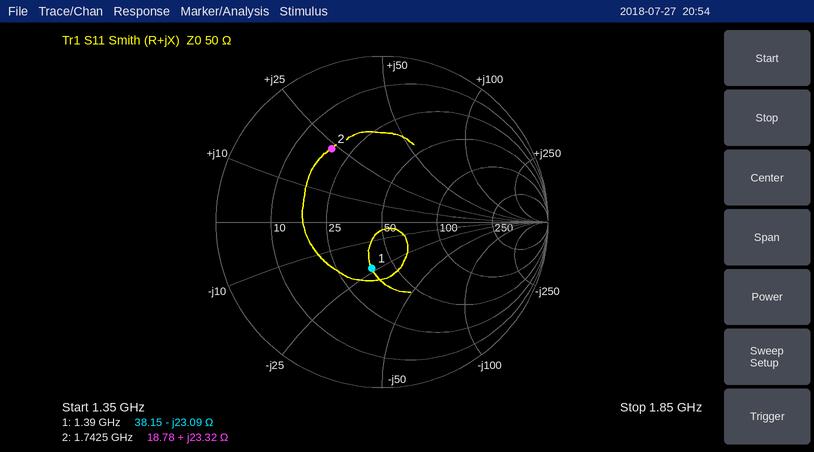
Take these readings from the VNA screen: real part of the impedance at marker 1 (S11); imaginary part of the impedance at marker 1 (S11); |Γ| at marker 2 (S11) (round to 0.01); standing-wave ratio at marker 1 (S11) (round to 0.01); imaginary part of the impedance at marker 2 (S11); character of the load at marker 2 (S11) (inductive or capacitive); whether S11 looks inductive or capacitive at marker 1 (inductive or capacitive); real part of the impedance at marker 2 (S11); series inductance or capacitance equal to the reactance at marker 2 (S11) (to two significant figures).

38.15 Ω
-23.09 Ω
0.54
1.80
+23.32 Ω
inductive
capacitive
18.78 Ω
2.1 nH
